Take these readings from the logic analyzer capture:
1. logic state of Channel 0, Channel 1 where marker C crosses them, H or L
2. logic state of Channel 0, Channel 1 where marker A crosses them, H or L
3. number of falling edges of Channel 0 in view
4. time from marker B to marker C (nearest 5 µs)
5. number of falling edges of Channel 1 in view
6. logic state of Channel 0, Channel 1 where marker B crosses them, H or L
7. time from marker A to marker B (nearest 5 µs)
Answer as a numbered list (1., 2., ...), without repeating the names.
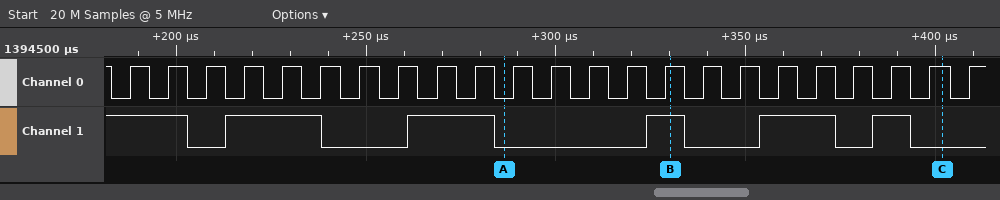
1. Channel 0=H, Channel 1=L
2. Channel 0=L, Channel 1=L
3. 23
4. 70 µs
5. 6
6. Channel 0=H, Channel 1=H
7. 45 µs
